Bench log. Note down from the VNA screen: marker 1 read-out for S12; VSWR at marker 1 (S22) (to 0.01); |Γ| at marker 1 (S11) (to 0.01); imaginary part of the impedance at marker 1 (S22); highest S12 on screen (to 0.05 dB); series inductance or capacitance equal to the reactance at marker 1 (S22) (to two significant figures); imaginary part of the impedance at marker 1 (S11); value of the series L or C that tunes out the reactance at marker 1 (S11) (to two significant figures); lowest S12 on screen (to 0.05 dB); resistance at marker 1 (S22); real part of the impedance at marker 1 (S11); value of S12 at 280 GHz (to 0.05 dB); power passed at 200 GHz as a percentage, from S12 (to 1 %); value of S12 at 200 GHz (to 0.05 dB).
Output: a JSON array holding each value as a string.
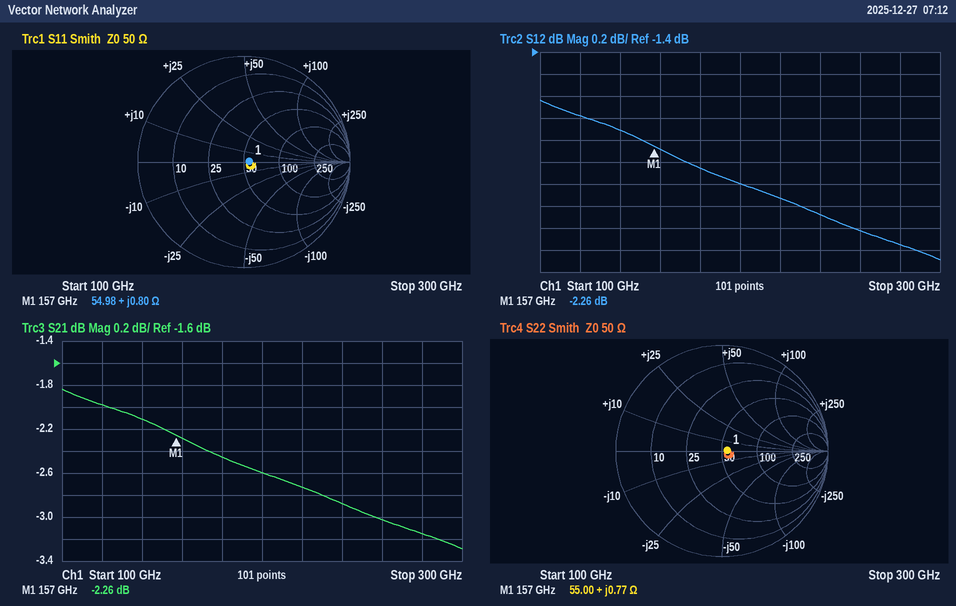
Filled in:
["-2.26 dB", "1.10", "0.05", "+0.77 Ω", "-1.85 dB", "780 fH", "+0.80 Ω", "1.3 pF", "-3.30 dB", "55.00 Ω", "54.98 Ω", "-3.15 dB", "55 %", "-2.60 dB"]
